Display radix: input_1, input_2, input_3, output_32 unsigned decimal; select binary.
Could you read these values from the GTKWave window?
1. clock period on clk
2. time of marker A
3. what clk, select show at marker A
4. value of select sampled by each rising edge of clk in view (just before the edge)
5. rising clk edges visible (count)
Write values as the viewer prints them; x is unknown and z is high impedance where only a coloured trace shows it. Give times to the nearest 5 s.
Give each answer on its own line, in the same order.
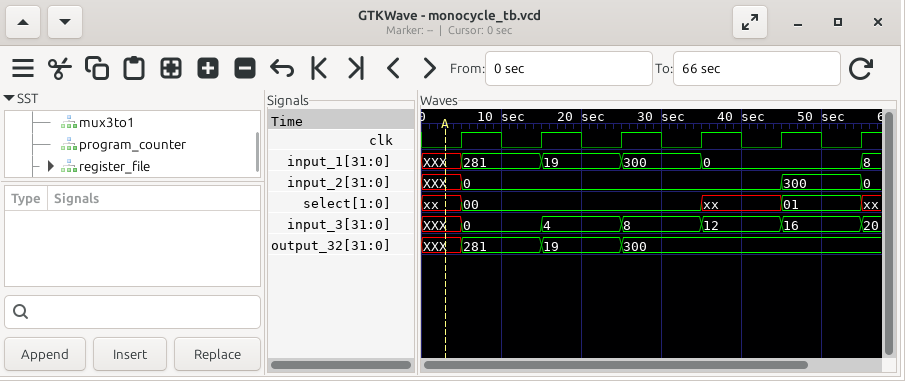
10 s
5 s
clk=0, select=xx
xx, 00, 00, 00, xx, 01
6
